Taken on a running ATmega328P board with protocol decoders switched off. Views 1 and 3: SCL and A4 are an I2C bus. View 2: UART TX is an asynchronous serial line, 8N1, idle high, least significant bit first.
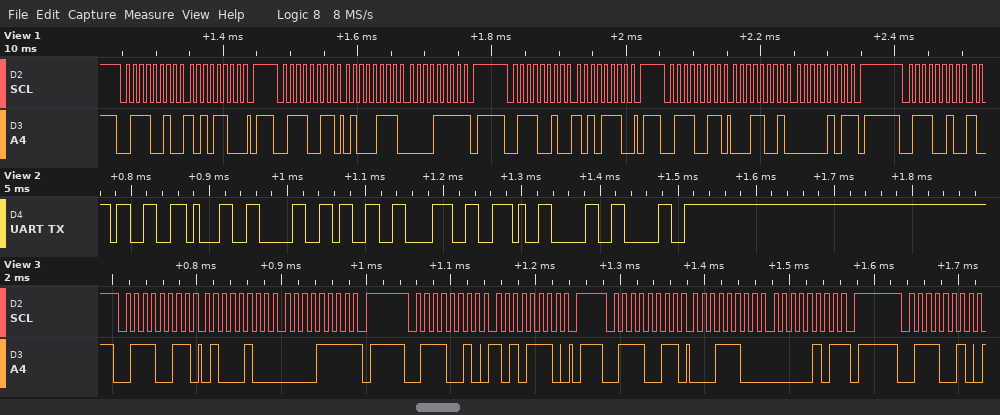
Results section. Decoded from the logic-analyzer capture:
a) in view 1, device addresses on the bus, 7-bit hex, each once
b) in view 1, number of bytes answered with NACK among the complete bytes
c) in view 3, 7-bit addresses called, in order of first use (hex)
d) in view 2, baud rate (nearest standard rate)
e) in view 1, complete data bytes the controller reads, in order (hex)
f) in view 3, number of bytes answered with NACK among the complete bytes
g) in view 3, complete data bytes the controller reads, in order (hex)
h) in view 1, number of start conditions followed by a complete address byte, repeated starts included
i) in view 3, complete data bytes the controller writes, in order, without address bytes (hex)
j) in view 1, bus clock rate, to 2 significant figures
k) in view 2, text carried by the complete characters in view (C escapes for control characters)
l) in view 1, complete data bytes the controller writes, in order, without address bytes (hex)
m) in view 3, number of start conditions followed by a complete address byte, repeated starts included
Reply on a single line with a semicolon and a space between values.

0x39; 2; 0x39; 115200 baud; 47 0F 19 05; 2; 44 0F 1C 05; 5; AE; 100 kHz; "31038.00"; AC AE; 4
